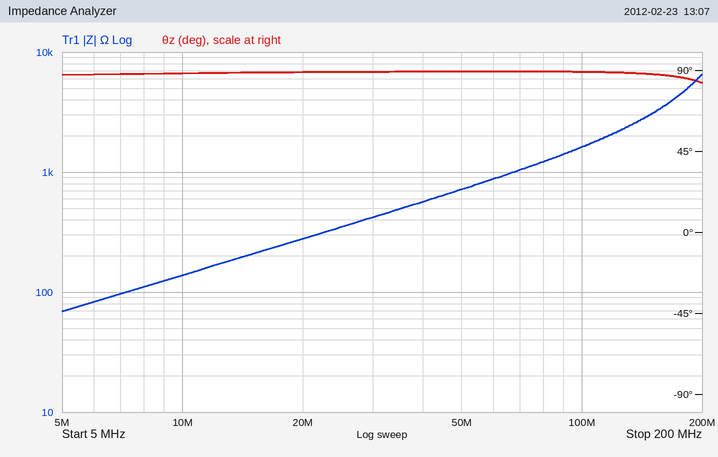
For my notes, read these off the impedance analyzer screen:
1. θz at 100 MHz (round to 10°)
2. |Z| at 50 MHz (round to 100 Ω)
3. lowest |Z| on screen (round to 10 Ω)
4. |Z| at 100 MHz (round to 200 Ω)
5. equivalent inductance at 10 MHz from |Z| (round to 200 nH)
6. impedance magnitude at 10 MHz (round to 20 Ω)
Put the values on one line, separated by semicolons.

90°; 700 Ω; 70 Ω; 1.6 kΩ; 2.2 µH; 140 Ω
